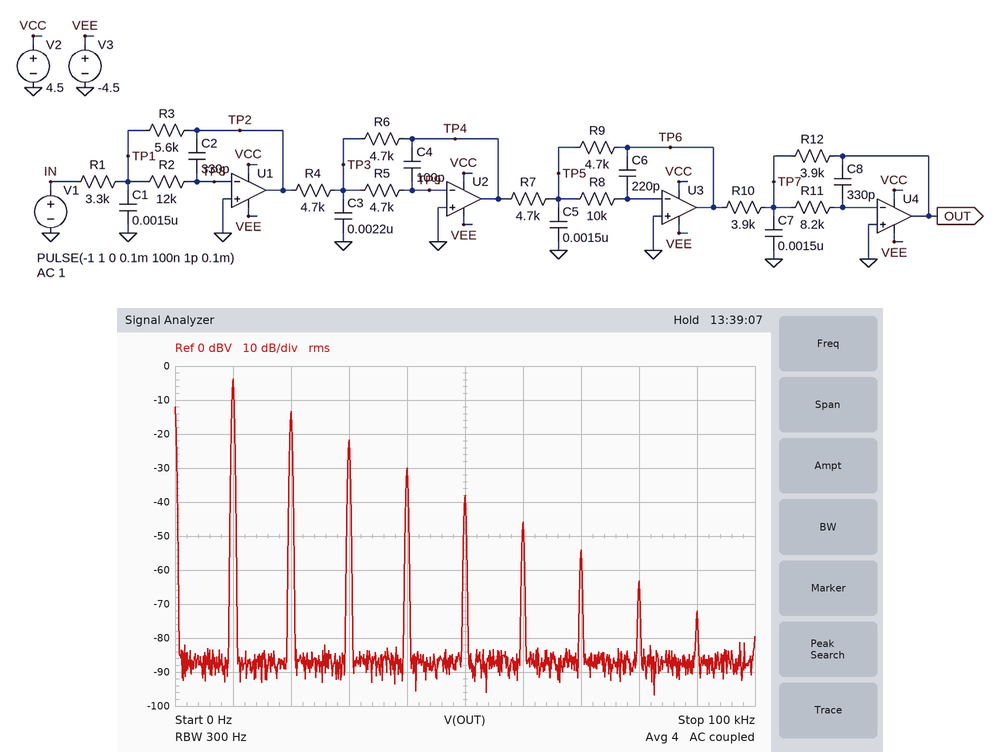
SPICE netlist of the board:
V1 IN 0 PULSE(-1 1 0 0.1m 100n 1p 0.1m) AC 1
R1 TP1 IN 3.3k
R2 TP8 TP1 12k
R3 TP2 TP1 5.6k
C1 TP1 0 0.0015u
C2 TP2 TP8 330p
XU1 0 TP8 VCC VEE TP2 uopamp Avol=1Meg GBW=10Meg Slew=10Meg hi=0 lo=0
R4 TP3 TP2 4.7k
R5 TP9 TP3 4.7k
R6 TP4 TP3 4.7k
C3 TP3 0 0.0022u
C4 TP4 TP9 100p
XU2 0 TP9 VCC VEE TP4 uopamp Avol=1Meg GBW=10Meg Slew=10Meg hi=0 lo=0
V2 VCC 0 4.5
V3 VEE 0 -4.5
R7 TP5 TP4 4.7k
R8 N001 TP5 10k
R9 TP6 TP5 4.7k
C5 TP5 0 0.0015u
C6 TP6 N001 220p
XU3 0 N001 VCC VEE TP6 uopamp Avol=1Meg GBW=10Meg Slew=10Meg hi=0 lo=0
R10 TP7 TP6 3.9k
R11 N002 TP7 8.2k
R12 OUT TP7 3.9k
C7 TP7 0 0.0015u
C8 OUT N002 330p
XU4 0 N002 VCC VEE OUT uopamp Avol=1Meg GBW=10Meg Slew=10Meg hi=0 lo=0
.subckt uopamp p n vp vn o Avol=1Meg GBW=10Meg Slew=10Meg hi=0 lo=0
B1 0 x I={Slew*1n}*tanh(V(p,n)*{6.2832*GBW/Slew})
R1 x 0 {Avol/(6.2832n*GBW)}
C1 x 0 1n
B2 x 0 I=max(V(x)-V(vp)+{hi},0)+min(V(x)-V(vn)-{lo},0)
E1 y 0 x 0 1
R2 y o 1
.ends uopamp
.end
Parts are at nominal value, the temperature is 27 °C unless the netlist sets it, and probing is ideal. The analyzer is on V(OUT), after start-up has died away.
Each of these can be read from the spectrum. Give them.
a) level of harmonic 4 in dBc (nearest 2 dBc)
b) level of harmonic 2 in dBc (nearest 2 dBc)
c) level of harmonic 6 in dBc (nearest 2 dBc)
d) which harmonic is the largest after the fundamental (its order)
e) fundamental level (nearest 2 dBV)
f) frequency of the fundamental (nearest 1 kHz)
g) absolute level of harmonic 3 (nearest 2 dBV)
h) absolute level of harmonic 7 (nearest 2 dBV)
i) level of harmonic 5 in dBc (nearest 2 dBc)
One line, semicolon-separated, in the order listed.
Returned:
-26 dBc; -10 dBc; -42 dBc; 2; -4 dBV; 10 kHz; -22 dBV; -54 dBV; -34 dBc
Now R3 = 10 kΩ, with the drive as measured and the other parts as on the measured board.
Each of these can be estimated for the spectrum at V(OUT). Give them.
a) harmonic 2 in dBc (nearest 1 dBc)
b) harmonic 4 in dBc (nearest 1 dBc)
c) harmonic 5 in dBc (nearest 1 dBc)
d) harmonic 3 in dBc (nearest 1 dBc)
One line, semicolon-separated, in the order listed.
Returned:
-11 dBc; -29 dBc; -37 dBc; -20 dBc
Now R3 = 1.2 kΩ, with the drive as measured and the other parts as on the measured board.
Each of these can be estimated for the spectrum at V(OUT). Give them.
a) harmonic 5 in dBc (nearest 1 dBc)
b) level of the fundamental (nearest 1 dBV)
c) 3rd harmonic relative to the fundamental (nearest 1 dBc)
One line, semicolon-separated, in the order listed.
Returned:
-27 dBc; -16 dBV; -14 dBc
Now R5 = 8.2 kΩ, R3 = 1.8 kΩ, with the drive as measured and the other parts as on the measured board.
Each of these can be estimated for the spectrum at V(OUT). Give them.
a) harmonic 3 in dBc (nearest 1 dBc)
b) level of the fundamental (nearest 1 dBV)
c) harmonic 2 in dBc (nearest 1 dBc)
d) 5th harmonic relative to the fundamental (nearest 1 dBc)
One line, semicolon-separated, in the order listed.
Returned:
-14 dBc; -13 dBV; -7 dBc; -29 dBc
